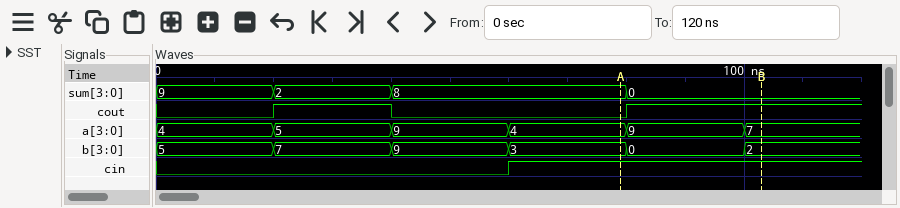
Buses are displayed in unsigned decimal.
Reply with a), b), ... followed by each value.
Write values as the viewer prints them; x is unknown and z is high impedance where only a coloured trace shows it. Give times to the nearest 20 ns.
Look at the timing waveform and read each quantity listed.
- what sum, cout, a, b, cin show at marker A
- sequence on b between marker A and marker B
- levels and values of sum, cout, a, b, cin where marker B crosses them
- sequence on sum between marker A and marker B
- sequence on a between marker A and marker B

a) sum=8, cout=0, a=4, b=3, cin=1
b) 3, 0, 2
c) sum=0, cout=1, a=7, b=2, cin=1
d) 8, 0
e) 4, 9, 7
